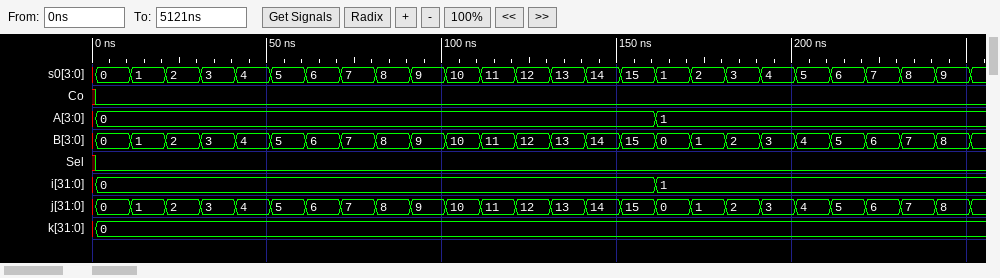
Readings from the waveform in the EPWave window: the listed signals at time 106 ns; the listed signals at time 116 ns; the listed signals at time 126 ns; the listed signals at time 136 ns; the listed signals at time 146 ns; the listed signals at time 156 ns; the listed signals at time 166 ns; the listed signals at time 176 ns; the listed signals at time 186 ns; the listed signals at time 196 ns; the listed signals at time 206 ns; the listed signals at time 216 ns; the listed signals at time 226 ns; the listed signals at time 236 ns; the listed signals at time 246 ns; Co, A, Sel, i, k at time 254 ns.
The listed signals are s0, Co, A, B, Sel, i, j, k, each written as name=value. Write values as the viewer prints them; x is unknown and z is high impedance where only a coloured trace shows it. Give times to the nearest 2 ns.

s0=10, Co=0, A=0, B=10, Sel=0, i=0, j=10, k=0
s0=11, Co=0, A=0, B=11, Sel=0, i=0, j=11, k=0
s0=12, Co=0, A=0, B=12, Sel=0, i=0, j=12, k=0
s0=13, Co=0, A=0, B=13, Sel=0, i=0, j=13, k=0
s0=14, Co=0, A=0, B=14, Sel=0, i=0, j=14, k=0
s0=15, Co=0, A=0, B=15, Sel=0, i=0, j=15, k=0
s0=1, Co=0, A=1, B=0, Sel=0, i=1, j=0, k=0
s0=2, Co=0, A=1, B=1, Sel=0, i=1, j=1, k=0
s0=3, Co=0, A=1, B=2, Sel=0, i=1, j=2, k=0
s0=4, Co=0, A=1, B=3, Sel=0, i=1, j=3, k=0
s0=5, Co=0, A=1, B=4, Sel=0, i=1, j=4, k=0
s0=6, Co=0, A=1, B=5, Sel=0, i=1, j=5, k=0
s0=7, Co=0, A=1, B=6, Sel=0, i=1, j=6, k=0
s0=8, Co=0, A=1, B=7, Sel=0, i=1, j=7, k=0
s0=9, Co=0, A=1, B=8, Sel=0, i=1, j=8, k=0
Co=0, A=1, Sel=0, i=1, k=0
